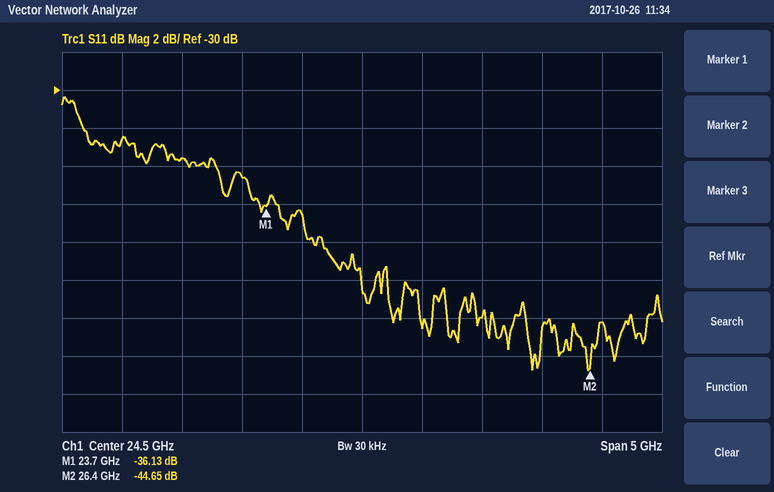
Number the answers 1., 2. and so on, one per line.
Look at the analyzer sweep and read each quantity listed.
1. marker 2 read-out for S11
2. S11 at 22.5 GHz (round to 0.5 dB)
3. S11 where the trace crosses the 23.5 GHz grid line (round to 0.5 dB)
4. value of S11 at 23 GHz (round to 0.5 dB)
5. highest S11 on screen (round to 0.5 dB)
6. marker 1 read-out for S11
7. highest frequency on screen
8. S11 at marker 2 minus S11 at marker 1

1. -44.65 dB
2. -32.5 dB
3. -34.5 dB
4. -33.5 dB
5. -30.5 dB
6. -36.13 dB
7. 27 GHz
8. -8.52 dB
